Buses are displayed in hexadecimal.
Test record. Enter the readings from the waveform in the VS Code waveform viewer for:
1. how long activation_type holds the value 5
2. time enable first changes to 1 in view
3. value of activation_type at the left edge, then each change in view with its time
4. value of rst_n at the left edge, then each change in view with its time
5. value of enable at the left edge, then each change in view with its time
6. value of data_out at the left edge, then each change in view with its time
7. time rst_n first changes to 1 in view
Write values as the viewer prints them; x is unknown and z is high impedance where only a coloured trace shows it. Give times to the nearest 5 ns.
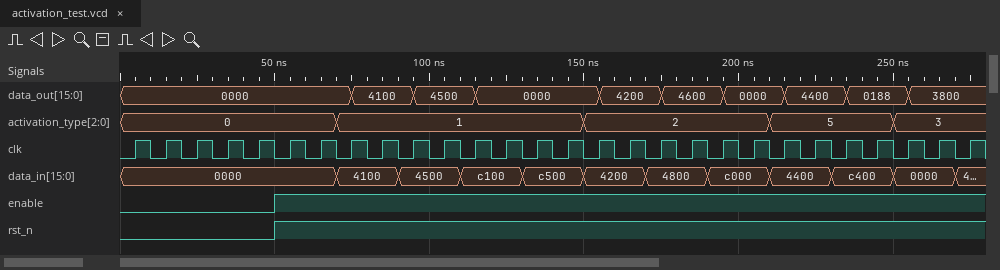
40 ns
50 ns
0, 1 at 70 ns, 2 at 150 ns, 5 at 210 ns, 3 at 250 ns
0, 1 at 50 ns
0, 1 at 50 ns
0000, 4100 at 75 ns, 4500 at 95 ns, 0000 at 115 ns, 4200 at 155 ns, 4600 at 175 ns, 0000 at 195 ns, 4400 at 215 ns, 0188 at 235 ns, 3800 at 255 ns
50 ns
